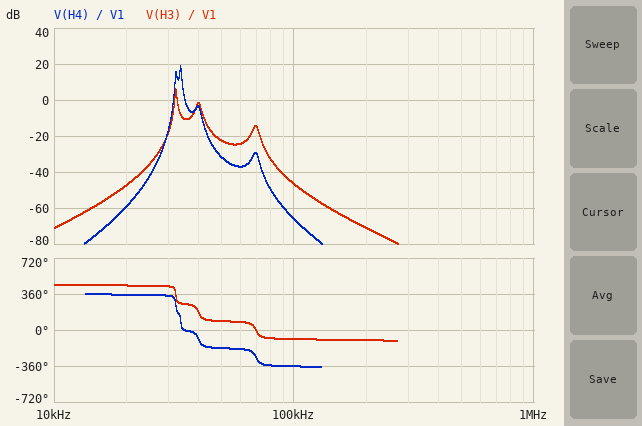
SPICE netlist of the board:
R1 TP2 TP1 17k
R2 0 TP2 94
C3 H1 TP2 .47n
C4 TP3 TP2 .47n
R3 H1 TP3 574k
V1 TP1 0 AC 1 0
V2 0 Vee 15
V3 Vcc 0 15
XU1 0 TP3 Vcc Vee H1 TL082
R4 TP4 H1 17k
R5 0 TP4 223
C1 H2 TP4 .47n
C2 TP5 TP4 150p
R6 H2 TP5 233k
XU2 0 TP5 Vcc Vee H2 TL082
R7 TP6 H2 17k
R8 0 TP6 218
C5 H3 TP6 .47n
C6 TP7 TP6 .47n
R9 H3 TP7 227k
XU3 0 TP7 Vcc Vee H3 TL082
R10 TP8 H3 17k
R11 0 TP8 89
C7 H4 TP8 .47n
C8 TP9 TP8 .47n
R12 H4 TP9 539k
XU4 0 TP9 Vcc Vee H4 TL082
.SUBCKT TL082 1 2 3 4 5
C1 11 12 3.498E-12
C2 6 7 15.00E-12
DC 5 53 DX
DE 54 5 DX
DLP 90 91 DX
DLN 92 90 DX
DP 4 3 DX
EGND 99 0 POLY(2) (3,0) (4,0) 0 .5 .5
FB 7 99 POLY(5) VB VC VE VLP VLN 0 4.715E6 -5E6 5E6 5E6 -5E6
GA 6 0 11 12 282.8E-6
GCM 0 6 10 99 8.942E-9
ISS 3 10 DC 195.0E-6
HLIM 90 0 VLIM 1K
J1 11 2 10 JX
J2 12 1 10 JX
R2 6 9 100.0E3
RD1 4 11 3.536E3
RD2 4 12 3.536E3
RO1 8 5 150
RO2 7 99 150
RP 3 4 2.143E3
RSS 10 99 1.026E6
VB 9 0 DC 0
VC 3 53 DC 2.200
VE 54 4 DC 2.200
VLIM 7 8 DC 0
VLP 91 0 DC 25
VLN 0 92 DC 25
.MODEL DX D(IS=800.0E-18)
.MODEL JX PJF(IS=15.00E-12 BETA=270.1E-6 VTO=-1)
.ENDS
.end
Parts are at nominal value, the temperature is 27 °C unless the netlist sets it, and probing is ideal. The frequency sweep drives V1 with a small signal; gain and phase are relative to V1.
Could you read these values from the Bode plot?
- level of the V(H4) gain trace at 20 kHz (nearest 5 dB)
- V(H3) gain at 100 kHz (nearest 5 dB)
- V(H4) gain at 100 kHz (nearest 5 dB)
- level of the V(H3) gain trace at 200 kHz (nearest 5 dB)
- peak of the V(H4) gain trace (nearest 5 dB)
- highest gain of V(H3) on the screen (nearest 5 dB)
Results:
-60 dB
-45 dB
-65 dB
-70 dB
20 dB
5 dB
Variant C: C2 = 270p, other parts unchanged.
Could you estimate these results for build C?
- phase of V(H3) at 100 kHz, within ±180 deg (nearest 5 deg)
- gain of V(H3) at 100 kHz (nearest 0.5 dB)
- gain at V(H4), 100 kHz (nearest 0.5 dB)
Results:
-95 deg
-49.5 dB
-69.0 dB
